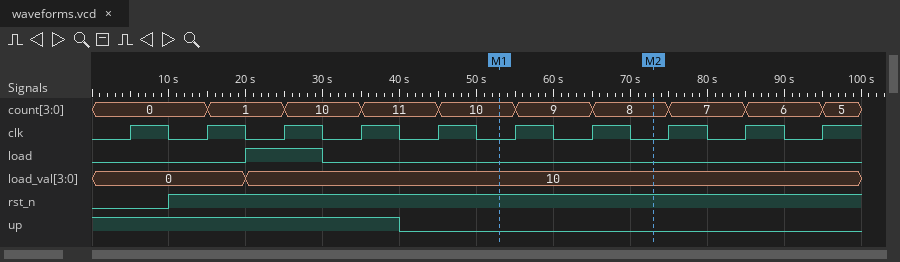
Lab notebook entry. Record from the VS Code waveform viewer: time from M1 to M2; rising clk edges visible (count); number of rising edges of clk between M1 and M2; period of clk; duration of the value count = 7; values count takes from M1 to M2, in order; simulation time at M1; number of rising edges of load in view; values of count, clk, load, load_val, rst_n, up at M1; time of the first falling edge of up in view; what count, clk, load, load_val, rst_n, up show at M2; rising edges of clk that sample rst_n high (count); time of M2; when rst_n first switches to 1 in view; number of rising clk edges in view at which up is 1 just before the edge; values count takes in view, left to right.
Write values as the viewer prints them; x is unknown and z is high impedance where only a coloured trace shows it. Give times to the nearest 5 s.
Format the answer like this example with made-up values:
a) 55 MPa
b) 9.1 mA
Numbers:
a) 20 s
b) 10
c) 2
d) 10 s
e) 10 s
f) 10, 9, 8
g) 55 s
h) 1
i) count=10, clk=0, load=0, load_val=10, rst_n=1, up=0
j) 40 s
k) count=8, clk=0, load=0, load_val=10, rst_n=1, up=0
l) 9
m) 75 s
n) 10 s
o) 4
p) 0, 1, 10, 11, 10, 9, 8, 7, 6, 5
